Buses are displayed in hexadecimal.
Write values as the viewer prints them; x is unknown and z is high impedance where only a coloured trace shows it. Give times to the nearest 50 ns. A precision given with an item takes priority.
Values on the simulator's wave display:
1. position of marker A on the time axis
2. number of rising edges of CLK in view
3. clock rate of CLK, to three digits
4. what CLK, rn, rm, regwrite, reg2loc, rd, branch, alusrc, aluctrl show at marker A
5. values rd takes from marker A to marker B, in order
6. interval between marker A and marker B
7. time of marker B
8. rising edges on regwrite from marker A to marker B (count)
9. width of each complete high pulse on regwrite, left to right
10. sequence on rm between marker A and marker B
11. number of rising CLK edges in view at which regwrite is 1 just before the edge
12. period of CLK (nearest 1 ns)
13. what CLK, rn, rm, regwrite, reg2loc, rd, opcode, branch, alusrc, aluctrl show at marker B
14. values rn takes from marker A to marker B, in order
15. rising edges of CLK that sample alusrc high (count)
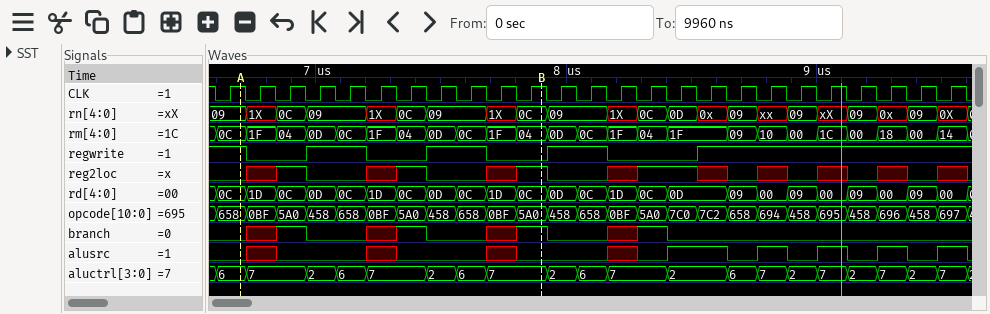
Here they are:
6700 ns
25
8.33 MHz
CLK=1, rn=09, rm=0C, regwrite=1, reg2loc=0, rd=0C, branch=0, alusrc=0, aluctrl=6
0C, 1D, 0C, 0D, 0C, 1D, 0C, 0D, 0C, 1D, 0C
1200 ns
7900 ns
2
250 ns, 250 ns, 250 ns
0C, 1F, 04, 0D, 0C, 1F, 04, 0D, 0C, 1F, 04
16
120 ns
CLK=1, rn=0C, rm=04, regwrite=0, reg2loc=1, rd=0C, opcode=5A0, branch=1, alusrc=0, aluctrl=7
09, 1X, 0C, 09, 1X, 0C, 09, 1X, 0C
6
